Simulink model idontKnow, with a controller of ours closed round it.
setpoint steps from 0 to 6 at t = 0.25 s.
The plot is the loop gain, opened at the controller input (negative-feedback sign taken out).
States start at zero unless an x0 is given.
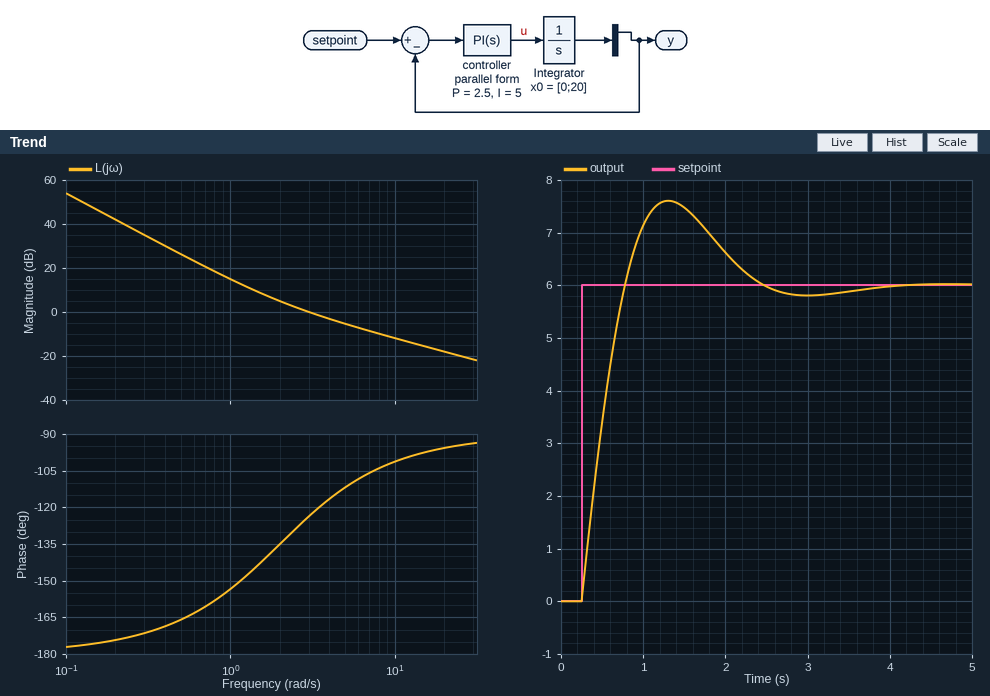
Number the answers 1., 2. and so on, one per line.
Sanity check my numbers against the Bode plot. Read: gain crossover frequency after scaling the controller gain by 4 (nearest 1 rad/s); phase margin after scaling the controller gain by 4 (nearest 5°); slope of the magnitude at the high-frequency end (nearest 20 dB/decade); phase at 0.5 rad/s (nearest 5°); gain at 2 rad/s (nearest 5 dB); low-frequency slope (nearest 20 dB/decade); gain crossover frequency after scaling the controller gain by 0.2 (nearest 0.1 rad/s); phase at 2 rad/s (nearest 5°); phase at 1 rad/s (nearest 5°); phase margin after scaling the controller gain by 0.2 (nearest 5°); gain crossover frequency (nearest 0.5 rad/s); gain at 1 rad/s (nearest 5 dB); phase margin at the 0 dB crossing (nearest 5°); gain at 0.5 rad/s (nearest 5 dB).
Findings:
1. 10 rad/s
2. 80°
3. -20 dB/decade
4. -165°
5. 5 dB
6. -40 dB/decade
7. 1.1 rad/s
8. -135°
9. -155°
10. 30°
11. 3.0 rad/s
12. 15 dB
13. 55°
14. 25 dB
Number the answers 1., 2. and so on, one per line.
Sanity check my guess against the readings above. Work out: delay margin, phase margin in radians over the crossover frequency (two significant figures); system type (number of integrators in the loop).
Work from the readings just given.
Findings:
1. 0.32 s
2. 2
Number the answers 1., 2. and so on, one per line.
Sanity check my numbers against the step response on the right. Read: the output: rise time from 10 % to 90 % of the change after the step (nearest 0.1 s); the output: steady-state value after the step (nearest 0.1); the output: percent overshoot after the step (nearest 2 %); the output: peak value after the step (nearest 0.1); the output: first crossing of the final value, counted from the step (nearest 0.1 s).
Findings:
1. 0.4 s
2. 6.0
3. 26 %
4. 7.6
5. 0.5 s
